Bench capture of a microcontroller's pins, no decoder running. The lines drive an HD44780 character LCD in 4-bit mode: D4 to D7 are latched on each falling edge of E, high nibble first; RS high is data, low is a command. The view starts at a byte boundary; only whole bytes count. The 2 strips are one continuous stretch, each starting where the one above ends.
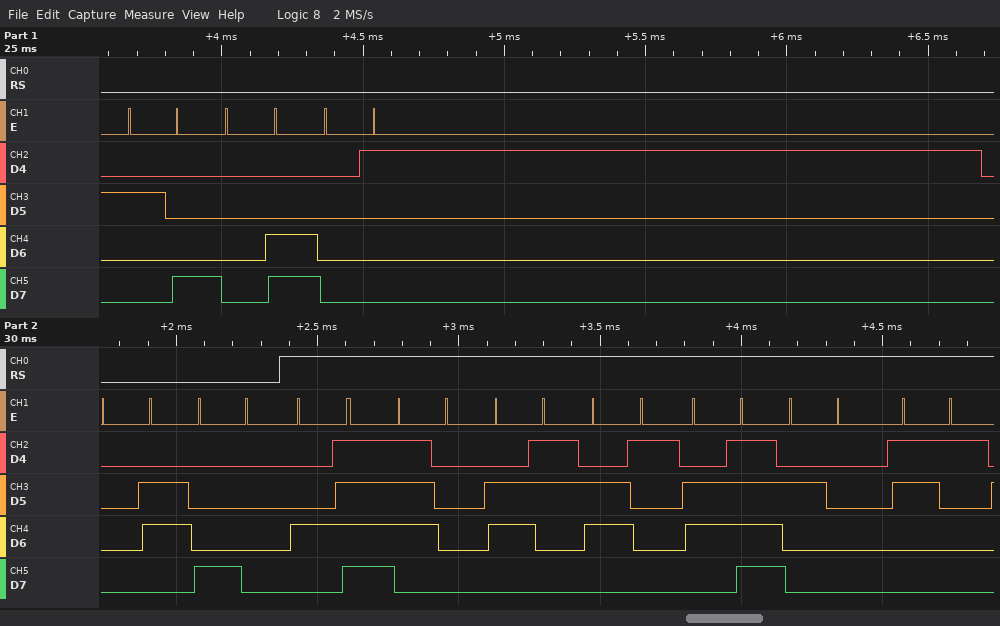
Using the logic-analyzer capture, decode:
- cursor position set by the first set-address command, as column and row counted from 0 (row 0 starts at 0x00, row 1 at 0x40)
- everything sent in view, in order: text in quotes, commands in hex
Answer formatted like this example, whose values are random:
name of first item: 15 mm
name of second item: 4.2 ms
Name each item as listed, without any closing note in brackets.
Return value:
cursor position set by the first set-address command, as column and row counted from 0: column 0, row 0
everything sent in view, in order: text in quotes, commands in hex: 0x28 0x0C 0x01 0x06 0x80 "Opcao 1"
